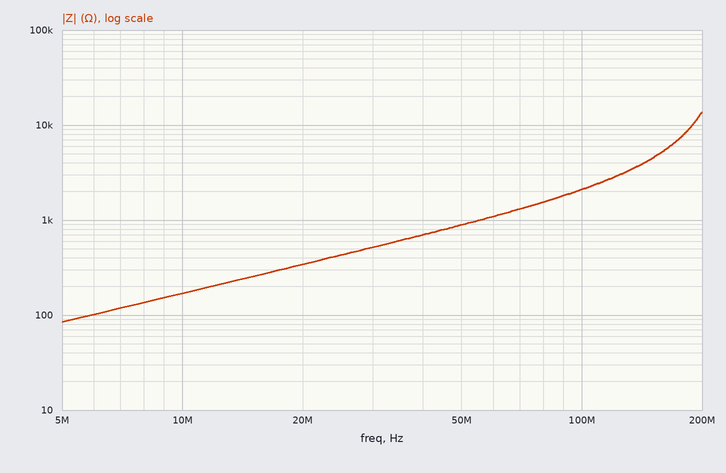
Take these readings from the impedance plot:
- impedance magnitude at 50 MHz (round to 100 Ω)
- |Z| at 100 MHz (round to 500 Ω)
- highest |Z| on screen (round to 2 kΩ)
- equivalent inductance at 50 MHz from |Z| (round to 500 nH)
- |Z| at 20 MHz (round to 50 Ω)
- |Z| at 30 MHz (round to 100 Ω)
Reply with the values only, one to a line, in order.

900 Ω
2.0 kΩ
14 kΩ
3.0 µH
350 Ω
500 Ω
